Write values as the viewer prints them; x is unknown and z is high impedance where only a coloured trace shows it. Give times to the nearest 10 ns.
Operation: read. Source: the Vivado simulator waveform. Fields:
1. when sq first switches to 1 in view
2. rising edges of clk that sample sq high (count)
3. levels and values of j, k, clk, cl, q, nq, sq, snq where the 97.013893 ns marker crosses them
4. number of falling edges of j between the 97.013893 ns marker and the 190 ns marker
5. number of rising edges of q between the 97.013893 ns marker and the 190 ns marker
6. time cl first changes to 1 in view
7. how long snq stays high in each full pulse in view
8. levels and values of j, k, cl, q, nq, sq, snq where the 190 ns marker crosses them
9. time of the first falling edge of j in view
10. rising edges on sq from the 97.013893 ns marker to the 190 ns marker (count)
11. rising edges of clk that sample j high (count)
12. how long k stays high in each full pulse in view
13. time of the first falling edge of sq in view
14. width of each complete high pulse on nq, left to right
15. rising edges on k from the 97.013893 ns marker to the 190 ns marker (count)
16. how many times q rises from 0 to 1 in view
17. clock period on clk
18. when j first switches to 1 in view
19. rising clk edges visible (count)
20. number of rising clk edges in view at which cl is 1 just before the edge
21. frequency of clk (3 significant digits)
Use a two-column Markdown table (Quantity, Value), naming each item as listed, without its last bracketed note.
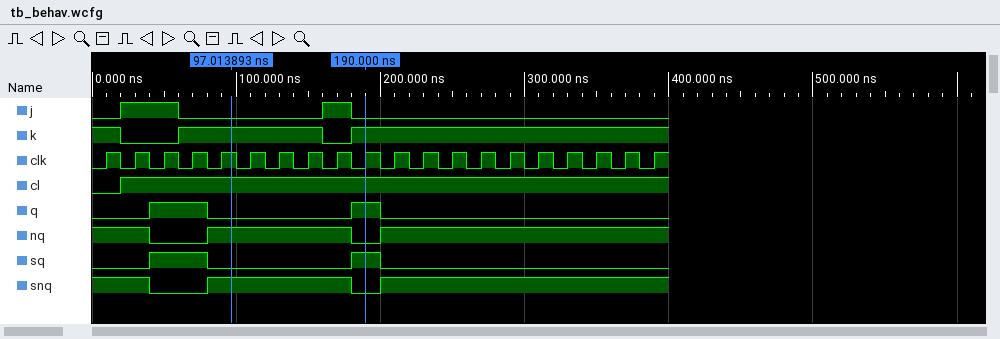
| Quantity | Value |
|---|---|
| when sq first switches to 1 in view | 40 ns |
| rising edges of clk that sample sq high | 3 |
| levels and values of j, k, clk, cl, q, nq, sq, snq where the 97.013893 ns marker crosses them | j=0, k=1, clk=1, cl=1, q=0, nq=1, sq=0, snq=1 |
| number of falling edges of j between the 97.013893 ns marker and the 190 ns marker | 1 |
| number of rising edges of q between the 97.013893 ns marker and the 190 ns marker | 1 |
| time cl first changes to 1 in view | 20 ns |
| how long snq stays high in each full pulse in view | 100 ns |
| levels and values of j, k, cl, q, nq, sq, snq where the 190 ns marker crosses them | j=0, k=1, cl=1, q=1, nq=0, sq=1, snq=0 |
| time of the first falling edge of j in view | 60 ns |
| rising edges on sq from the 97.013893 ns marker to the 190 ns marker | 1 |
| rising edges of clk that sample j high | 3 |
| how long k stays high in each full pulse in view | 100 ns |
| time of the first falling edge of sq in view | 80 ns |
| width of each complete high pulse on nq, left to right | 100 ns |
| rising edges on k from the 97.013893 ns marker to the 190 ns marker | 1 |
| how many times q rises from 0 to 1 in view | 2 |
| clock period on clk | 20 ns |
| when j first switches to 1 in view | 20 ns |
| rising clk edges visible | 20 |
| number of rising clk edges in view at which cl is 1 just before the edge | 19 |
| frequency of clk | 50.0 MHz |
